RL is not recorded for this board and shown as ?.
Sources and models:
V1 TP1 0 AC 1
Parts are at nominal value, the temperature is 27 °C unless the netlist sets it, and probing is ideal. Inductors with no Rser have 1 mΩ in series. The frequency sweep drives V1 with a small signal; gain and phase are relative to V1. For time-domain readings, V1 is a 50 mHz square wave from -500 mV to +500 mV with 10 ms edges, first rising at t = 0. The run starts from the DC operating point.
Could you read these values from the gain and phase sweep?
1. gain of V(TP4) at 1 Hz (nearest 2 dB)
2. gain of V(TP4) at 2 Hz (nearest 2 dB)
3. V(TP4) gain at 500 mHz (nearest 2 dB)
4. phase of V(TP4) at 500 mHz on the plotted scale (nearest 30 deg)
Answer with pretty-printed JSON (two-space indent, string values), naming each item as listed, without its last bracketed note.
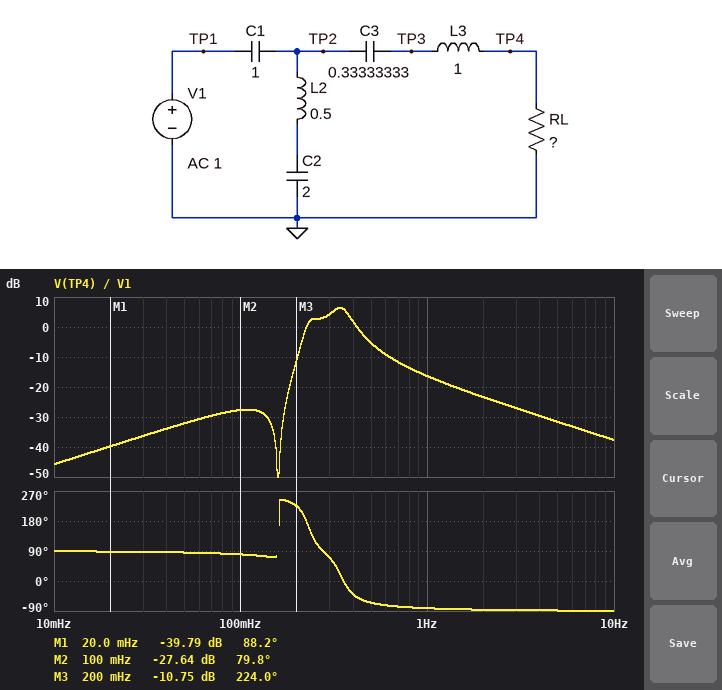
{
  "gain of V(TP4) at 1 Hz": "-16 dB",
  "gain of V(TP4) at 2 Hz": "-24 dB",
  "V(TP4) gain at 500 mHz": "-6 dB",
  "phase of V(TP4) at 500 mHz on the plotted scale": "-60 deg"
}
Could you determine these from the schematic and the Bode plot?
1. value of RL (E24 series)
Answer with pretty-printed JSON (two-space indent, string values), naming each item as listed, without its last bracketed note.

{
  "value of RL": "0.82 Ω"
}
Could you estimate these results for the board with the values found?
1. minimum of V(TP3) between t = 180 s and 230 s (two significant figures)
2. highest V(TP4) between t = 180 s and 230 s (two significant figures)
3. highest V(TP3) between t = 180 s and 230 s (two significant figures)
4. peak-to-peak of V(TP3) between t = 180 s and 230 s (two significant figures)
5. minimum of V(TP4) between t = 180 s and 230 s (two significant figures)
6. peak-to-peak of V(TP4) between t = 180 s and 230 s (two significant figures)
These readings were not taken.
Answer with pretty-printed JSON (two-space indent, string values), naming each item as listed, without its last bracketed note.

{
  "minimum of V(TP3) between t = 180 s and 230 s": "-1.1 V",
  "highest V(TP4) between t = 180 s and 230 s": "380 mV",
  "highest V(TP3) between t = 180 s and 230 s": "1.1 V",
  "peak-to-peak of V(TP3) between t = 180 s and 230 s": "2.2 V",
  "minimum of V(TP4) between t = 180 s and 230 s": "-380 mV",
  "peak-to-peak of V(TP4) between t = 180 s and 230 s": "760 mV"
}
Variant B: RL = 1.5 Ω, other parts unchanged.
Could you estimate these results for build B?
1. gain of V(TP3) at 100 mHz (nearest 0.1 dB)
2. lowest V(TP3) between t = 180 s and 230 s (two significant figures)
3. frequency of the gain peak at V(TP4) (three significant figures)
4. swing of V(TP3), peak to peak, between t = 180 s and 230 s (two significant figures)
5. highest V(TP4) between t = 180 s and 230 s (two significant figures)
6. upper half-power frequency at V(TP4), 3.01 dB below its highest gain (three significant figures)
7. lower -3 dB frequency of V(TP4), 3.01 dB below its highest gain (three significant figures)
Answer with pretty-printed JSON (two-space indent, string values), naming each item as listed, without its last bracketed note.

{
  "gain of V(TP3) at 100 mHz": "-22.0 dB",
  "lowest V(TP3) between t = 180 s and 230 s": "-900 mV",
  "frequency of the gain peak at V(TP4)": "290 mHz",
  "swing of V(TP3), peak to peak, between t = 180 s and 230 s": "1.8 V",
  "highest V(TP4) between t = 180 s and 230 s": "450 mV",
  "upper half-power frequency at V(TP4), 3.01 dB below its highest gain": "365 mHz",
  "lower -3 dB frequency of V(TP4), 3.01 dB below its highest gain": "247 mHz"
}
